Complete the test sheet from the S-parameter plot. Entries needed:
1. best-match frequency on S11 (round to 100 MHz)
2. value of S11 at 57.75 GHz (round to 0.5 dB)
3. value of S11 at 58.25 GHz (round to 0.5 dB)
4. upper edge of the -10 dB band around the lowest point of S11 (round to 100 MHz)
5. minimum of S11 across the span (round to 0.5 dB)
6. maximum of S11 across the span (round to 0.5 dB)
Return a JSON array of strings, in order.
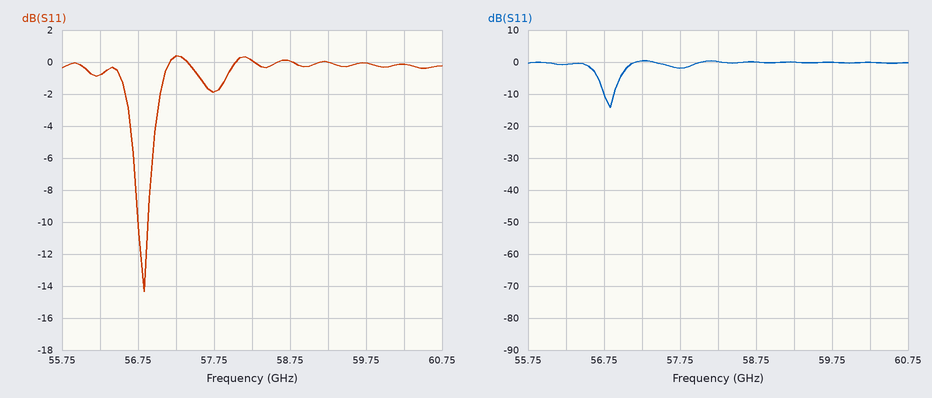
["56.8 GHz", "-2.0 dB", "0.0 dB", "56.9 GHz", "-14.5 dB", "0.5 dB"]
